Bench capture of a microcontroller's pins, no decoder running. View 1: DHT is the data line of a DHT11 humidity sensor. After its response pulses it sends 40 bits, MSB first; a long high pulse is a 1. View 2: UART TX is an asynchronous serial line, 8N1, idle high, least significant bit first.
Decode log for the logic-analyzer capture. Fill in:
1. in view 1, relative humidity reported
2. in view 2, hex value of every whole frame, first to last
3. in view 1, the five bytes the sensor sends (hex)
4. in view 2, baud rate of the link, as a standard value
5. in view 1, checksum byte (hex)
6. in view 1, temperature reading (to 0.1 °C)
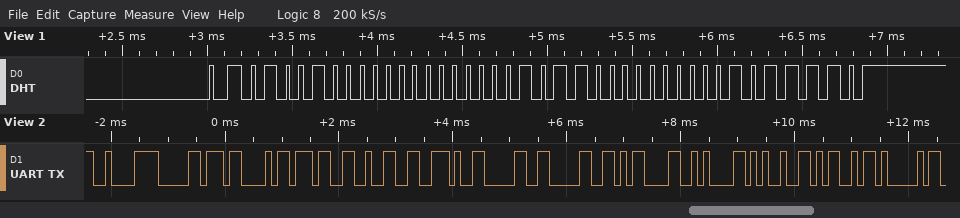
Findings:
72 %
C2 B0 43 37 32 2E 30 30 0D 0A 25 4D 41
48 00 16 00 5E
9600 baud
0x5E
22.0 °C
